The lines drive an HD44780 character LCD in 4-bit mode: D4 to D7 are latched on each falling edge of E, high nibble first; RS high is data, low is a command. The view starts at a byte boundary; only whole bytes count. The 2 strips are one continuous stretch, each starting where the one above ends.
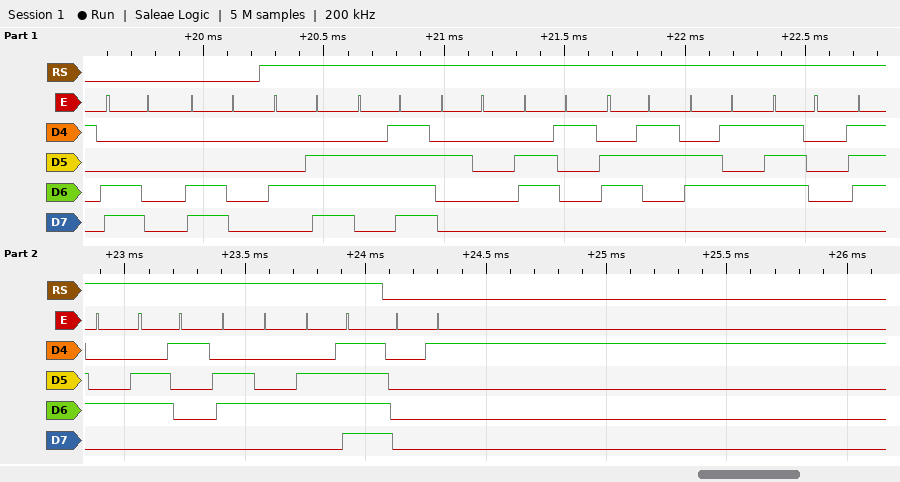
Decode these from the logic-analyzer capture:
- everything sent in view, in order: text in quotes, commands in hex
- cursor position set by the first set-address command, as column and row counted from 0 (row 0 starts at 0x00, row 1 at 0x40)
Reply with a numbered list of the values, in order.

1. 0xC0 0xC0 "No aceptado" 0x01
2. column 0, row 1
